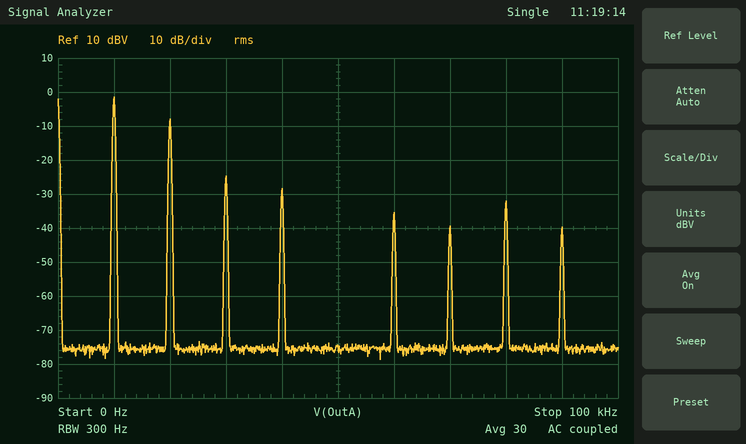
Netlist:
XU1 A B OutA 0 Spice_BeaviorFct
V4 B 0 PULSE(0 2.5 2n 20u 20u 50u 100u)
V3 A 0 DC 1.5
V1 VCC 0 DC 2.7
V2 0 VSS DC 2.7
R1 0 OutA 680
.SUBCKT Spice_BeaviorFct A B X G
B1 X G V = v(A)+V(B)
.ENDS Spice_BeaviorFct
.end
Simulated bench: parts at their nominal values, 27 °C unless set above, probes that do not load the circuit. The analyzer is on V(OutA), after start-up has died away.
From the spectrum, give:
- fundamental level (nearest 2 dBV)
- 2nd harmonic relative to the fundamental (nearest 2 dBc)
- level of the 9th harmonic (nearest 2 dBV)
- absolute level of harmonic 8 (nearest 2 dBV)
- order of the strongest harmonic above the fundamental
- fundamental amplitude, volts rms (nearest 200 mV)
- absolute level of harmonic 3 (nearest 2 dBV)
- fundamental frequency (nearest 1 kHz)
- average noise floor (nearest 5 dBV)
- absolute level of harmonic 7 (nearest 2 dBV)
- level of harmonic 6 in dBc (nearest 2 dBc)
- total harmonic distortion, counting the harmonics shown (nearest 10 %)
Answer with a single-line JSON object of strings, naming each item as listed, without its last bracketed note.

{"fundamental level": "-2 dBV", "2nd harmonic relative to the fundamental": "-6 dBc", "level of the 9th harmonic": "-40 dBV", "absolute level of harmonic 8": "-32 dBV", "order of the strongest harmonic above the fundamental": "2", "fundamental amplitude, volts rms": "800 mV", "absolute level of harmonic 3": "-24 dBV", "fundamental frequency": "10 kHz", "average noise floor": "-75 dBV", "absolute level of harmonic 7": "-40 dBV", "level of harmonic 6 in dBc": "-34 dBc", "total harmonic distortion, counting the harmonics shown": "50 %"}
